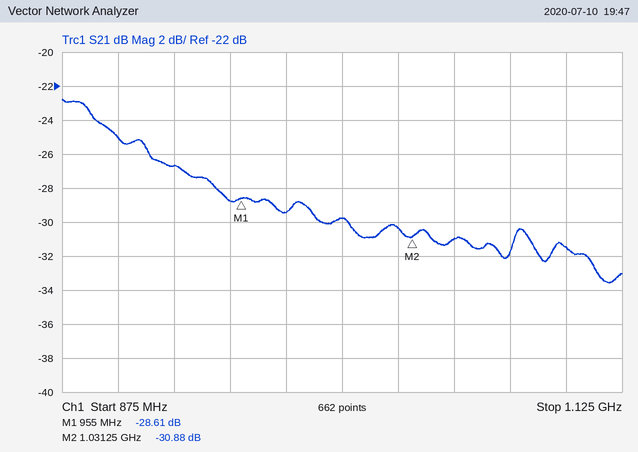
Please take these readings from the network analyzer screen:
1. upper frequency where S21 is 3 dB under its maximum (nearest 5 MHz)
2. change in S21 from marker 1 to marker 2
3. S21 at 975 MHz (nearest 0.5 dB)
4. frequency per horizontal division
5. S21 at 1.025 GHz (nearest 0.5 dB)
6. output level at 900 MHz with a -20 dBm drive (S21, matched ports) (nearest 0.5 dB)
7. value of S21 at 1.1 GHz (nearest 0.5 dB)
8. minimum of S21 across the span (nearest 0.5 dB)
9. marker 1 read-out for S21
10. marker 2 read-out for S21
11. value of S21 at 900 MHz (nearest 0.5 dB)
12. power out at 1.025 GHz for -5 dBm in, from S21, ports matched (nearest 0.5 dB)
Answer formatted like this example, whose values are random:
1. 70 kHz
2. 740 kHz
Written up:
1. 915 MHz
2. -2.27 dB
3. -29.5 dB
4. 25 MHz
5. -30.5 dB
6. -45.0 dBm
7. -31.5 dB
8. -33.5 dB
9. -28.61 dB
10. -30.88 dB
11. -25.0 dB
12. -35.5 dBm
